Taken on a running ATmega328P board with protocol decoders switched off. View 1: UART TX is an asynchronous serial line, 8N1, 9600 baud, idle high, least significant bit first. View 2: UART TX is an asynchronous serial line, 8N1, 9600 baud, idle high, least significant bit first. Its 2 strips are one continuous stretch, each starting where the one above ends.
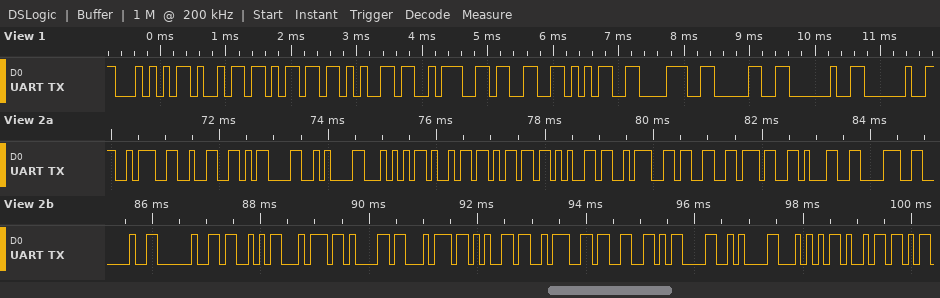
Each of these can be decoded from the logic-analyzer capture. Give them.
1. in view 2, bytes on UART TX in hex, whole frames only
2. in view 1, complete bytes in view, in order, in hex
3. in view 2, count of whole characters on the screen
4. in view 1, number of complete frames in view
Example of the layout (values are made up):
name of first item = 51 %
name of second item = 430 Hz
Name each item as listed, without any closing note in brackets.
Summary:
in view 2, bytes on UART TX in hex, whole frames only = 3A 32 0D 0A 54 69 6D 65 3A 33 37 31 38 20 20 53 74 61 74 65 3A 33 0D 0A 54 69
in view 1, complete bytes in view, in order, in hex = 54 69 6D 65 3A 33 35 38 30 20 20
in view 2, count of whole characters on the screen = 26
in view 1, number of complete frames in view = 11
